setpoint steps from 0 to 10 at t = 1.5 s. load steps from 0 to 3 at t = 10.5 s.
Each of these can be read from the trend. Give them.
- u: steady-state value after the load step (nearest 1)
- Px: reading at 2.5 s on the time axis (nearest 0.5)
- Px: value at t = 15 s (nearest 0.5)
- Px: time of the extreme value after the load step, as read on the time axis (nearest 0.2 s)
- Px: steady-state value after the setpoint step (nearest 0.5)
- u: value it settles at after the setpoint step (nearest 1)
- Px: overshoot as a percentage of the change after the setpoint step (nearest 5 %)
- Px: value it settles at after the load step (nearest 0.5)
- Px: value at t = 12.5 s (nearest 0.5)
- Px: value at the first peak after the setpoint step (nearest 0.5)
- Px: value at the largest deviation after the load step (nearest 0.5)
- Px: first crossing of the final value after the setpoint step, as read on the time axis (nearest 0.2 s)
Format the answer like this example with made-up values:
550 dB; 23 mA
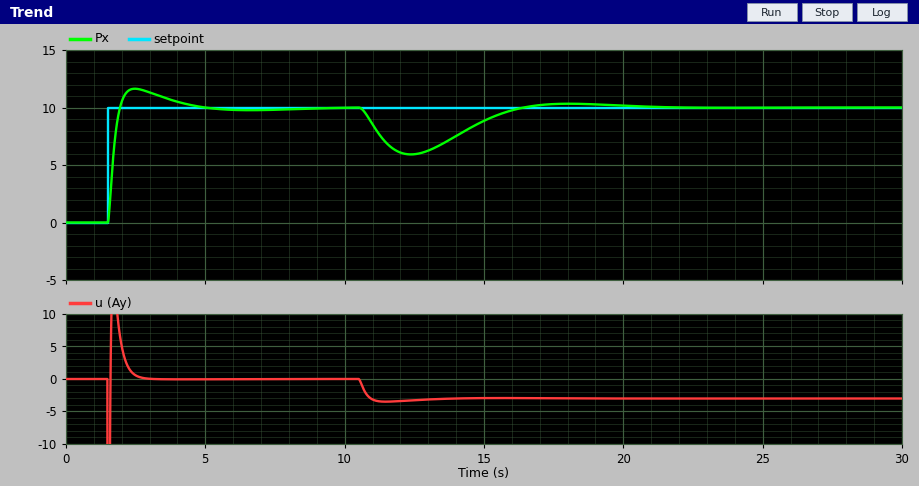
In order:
-3; 11.5; 9.0; 12.4 s; 10.0; 0; 15 %; 10.0; 6.0; 11.5; 6.0; 2.0 s
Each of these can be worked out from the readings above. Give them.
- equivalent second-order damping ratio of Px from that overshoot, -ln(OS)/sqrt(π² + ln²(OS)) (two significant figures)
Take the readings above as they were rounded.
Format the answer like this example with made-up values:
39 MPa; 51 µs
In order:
0.52
